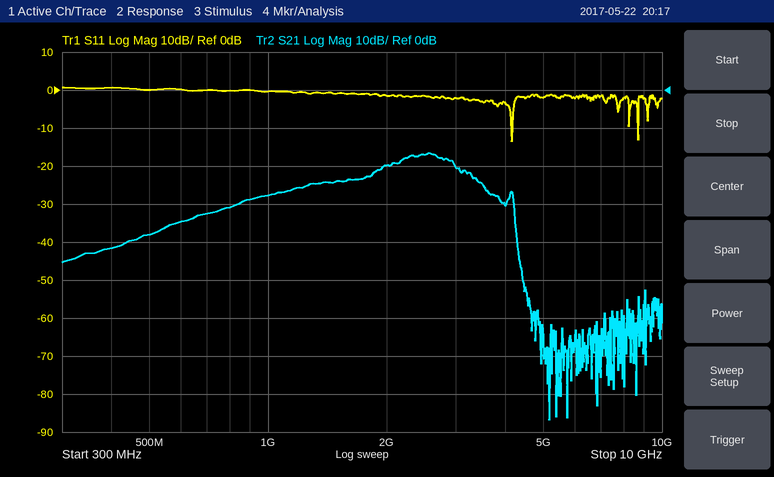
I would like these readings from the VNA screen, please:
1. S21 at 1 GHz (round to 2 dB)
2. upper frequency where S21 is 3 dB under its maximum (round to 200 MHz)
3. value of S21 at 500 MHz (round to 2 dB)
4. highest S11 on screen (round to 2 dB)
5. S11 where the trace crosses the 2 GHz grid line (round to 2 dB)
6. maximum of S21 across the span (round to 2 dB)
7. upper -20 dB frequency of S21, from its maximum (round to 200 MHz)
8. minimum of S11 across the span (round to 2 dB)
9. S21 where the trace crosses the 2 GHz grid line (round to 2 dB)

-28 dB
3.0 GHz
-38 dB
0 dB
-2 dB
-16 dB
4.2 GHz
-14 dB
-20 dB
